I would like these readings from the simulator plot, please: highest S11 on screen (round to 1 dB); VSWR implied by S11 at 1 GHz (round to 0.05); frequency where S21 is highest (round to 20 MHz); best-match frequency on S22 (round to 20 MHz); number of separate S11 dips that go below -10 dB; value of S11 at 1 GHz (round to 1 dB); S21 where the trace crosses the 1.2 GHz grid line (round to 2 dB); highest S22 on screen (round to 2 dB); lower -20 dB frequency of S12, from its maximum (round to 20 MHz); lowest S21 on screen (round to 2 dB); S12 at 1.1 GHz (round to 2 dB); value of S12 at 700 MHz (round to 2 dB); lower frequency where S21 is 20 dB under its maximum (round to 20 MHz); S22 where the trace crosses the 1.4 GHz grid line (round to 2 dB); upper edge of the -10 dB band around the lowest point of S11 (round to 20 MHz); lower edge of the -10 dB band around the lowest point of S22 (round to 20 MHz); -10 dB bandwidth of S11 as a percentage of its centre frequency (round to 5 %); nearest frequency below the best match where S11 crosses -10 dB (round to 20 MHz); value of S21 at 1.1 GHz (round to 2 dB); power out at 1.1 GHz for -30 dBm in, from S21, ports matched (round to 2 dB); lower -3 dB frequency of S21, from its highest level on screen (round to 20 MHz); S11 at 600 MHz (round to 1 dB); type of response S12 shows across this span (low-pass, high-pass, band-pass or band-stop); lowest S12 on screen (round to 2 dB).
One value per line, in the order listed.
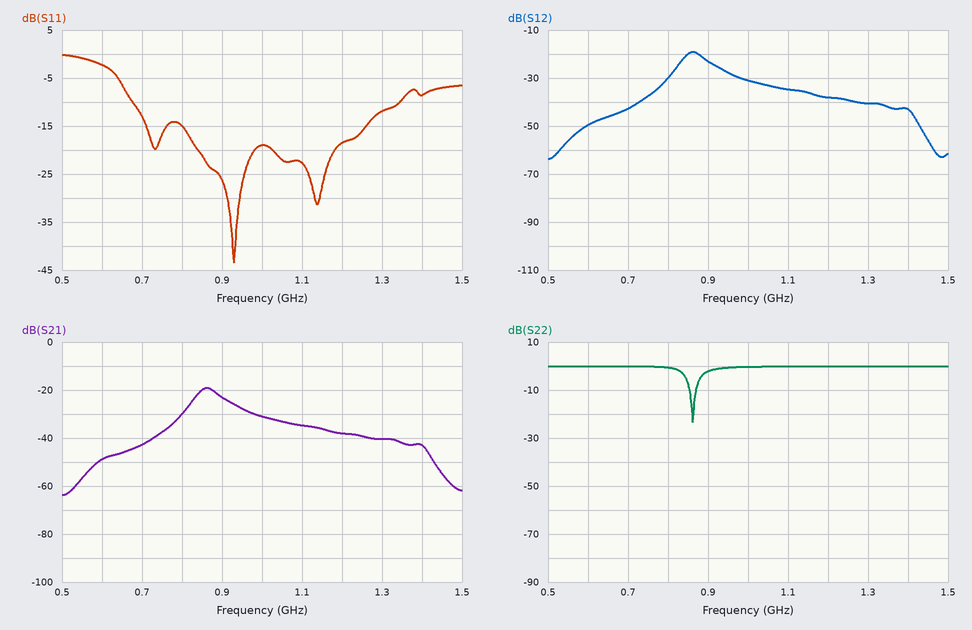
0 dB
1.25
860 MHz
860 MHz
3
-19 dB
-38 dB
0 dB
740 MHz
-64 dB
-34 dB
-42 dB
740 MHz
0 dB
1.34 GHz
860 MHz
65 %
680 MHz
-34 dB
-64 dBm
840 MHz
-2 dB
band-pass
-64 dB
